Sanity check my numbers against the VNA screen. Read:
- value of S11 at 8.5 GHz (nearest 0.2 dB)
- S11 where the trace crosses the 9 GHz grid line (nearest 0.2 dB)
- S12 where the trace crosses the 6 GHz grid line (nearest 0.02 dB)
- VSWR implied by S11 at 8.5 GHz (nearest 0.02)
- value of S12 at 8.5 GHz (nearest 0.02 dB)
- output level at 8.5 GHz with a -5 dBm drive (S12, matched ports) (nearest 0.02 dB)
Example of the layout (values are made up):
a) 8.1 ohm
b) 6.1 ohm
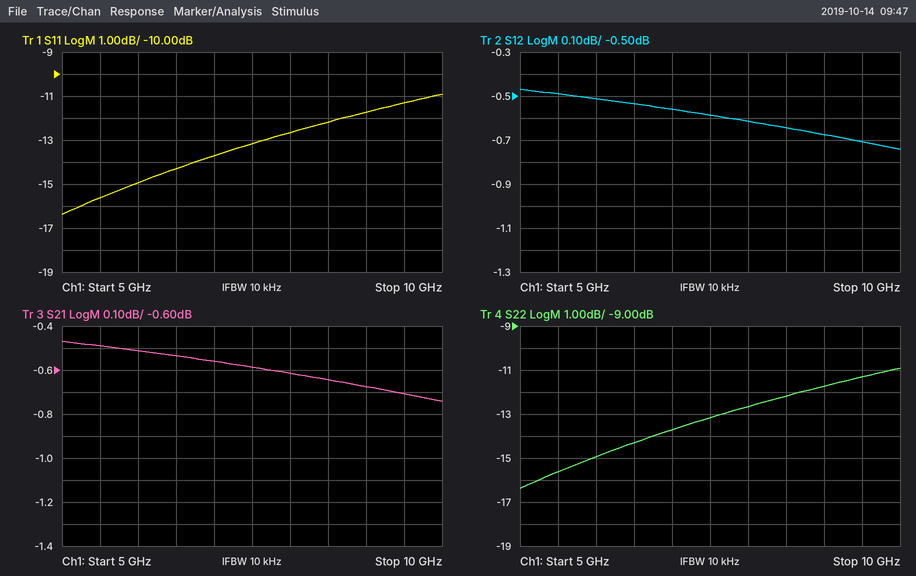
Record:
a) -12.2 dB
b) -11.8 dB
c) -0.52 dB
d) 1.66
e) -0.64 dB
f) -5.64 dBm
